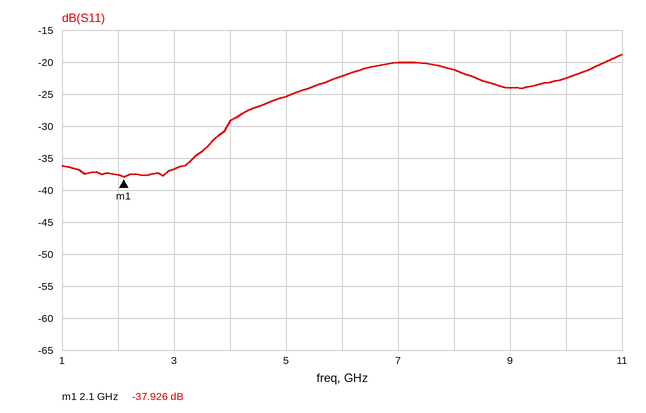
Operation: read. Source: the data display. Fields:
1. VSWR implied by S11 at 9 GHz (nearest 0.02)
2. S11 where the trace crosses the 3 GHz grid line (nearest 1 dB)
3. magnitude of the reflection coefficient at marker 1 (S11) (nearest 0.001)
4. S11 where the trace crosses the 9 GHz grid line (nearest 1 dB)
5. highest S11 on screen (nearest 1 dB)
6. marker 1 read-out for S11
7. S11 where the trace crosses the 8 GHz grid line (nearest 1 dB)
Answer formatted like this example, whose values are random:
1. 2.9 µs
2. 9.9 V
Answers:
1. 1.14
2. -37 dB
3. 0.013
4. -24 dB
5. -19 dB
6. -37.926 dB
7. -21 dB
